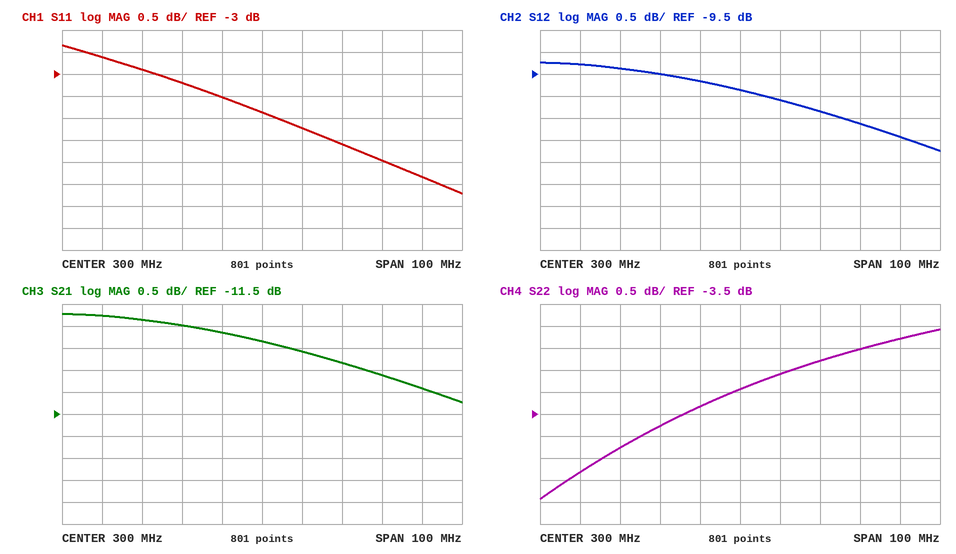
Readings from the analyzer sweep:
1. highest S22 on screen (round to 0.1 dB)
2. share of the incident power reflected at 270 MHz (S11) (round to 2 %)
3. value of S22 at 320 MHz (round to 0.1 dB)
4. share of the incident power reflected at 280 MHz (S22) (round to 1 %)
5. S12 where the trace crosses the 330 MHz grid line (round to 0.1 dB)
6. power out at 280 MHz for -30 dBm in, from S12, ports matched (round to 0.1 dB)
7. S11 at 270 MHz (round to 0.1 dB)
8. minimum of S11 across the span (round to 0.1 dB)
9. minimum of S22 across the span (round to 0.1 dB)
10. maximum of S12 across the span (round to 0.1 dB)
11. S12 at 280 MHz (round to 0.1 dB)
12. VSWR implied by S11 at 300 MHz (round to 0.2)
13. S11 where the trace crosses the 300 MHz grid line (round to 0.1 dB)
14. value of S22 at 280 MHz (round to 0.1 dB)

-1.6 dB
52 %
-2.3 dB
42 %
-10.6 dB
-39.5 dBm
-2.9 dB
-5.7 dB
-5.4 dB
-9.2 dB
-9.5 dB
4.6
-3.9 dB
-3.8 dB
